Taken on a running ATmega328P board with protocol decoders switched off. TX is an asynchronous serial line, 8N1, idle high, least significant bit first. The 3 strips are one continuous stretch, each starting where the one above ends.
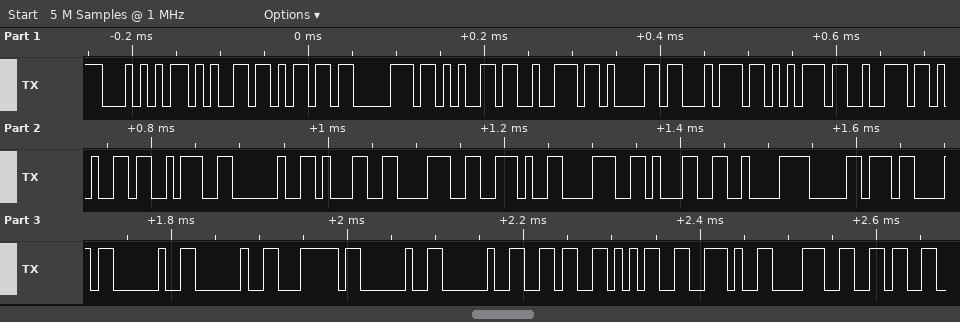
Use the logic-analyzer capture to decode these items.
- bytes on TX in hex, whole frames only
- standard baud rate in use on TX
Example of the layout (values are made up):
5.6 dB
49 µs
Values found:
54 65 6D 70 65 72 61 74 75 72 65 3A 20 31 38 2E 38 31 C2 B0 43 20 20 7C 20 20 36 35 2E 38 36
115200 baud
